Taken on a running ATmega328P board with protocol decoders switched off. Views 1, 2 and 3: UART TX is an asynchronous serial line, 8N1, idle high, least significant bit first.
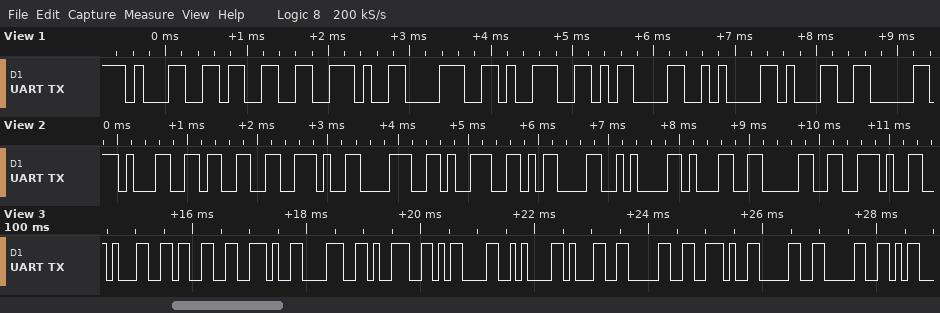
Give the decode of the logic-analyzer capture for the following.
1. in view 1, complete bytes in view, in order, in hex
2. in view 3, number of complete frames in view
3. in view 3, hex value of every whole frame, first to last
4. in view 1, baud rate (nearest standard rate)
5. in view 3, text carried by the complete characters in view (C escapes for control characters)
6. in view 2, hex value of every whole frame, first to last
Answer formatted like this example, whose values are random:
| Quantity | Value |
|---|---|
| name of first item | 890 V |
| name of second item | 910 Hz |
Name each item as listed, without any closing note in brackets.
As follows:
| Quantity | Value |
|---|---|
| in view 1, complete bytes in view, in order, in hex | 0x31 0x33 0x2E 0x38 0x39 0x0D 0x0A 0x31 |
| in view 3, number of complete frames in view | 12 |
| in view 3, hex value of every whole frame, first to last | 31 33 2E 38 39 0D 0A 31 30 2E 30 30 |
| in view 1, baud rate | 9600 baud |
| in view 3, text carried by the complete characters in view | "13.89\r\n10.00" |
| in view 2, hex value of every whole frame, first to last | 31 33 2E 38 39 0D 0A 31 30 2E |
